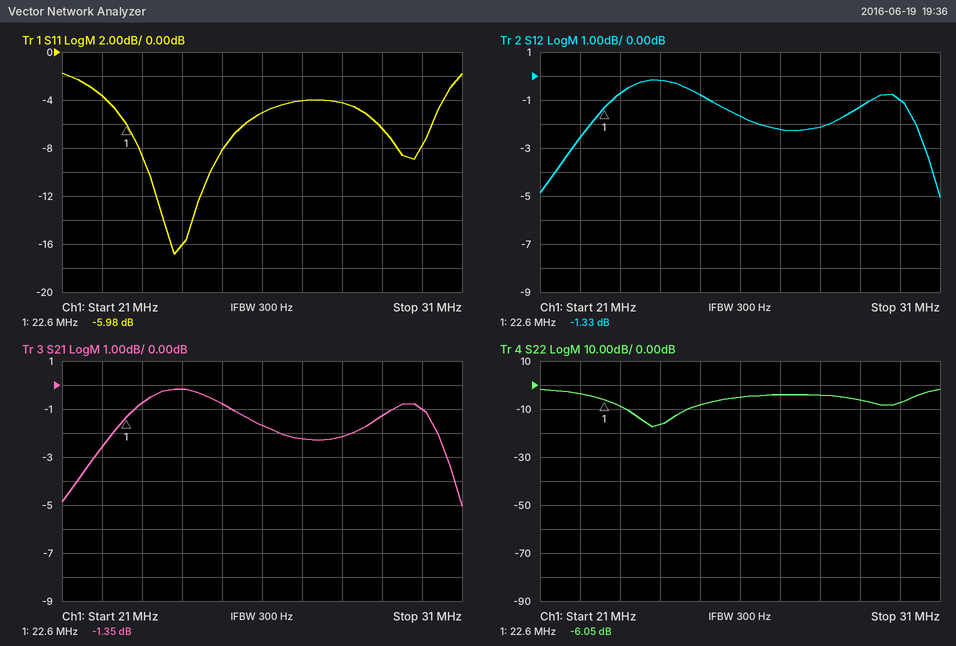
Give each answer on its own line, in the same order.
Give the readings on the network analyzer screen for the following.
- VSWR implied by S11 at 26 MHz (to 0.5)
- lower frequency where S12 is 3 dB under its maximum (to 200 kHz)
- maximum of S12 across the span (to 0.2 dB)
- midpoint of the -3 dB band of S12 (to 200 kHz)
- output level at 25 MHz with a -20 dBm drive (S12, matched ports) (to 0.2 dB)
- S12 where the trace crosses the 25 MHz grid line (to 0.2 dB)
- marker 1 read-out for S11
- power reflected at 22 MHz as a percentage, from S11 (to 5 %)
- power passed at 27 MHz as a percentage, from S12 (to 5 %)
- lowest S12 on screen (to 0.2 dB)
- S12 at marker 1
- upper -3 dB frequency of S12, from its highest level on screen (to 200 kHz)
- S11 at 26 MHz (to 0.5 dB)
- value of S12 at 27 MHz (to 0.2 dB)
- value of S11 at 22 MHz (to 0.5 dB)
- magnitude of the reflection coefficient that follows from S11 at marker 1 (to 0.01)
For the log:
3.5
21.8 MHz
-0.2 dB
26.2 MHz
-20.8 dBm
-0.8 dB
-5.98 dB
45 %
60 %
-5.0 dB
-1.33 dB
30.6 MHz
-5.0 dB
-2.2 dB
-3.5 dB
0.50
